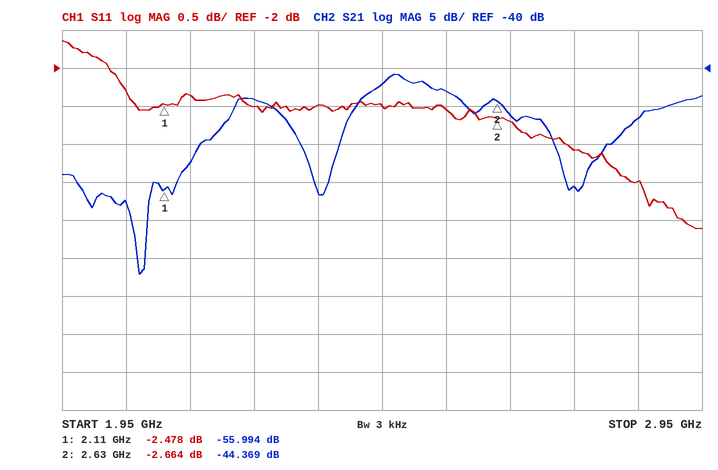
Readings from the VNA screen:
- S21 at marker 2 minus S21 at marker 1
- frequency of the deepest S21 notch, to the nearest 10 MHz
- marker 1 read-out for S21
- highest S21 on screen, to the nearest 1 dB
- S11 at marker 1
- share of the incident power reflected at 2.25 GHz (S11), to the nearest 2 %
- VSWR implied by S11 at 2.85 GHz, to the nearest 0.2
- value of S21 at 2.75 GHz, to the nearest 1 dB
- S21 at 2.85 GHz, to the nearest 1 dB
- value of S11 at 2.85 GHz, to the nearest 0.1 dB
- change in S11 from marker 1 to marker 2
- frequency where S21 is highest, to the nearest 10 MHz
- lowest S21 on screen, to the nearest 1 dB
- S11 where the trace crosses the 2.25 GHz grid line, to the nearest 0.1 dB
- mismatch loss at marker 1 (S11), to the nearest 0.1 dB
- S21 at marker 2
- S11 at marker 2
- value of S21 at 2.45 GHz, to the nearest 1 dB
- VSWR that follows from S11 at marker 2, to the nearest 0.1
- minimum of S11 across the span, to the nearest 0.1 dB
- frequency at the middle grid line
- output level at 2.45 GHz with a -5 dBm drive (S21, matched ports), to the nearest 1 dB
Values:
11.625 dB
2.07 GHz
-55.994 dB
-41 dB
-2.478 dB
56 %
5.0
-56 dB
-47 dB
-3.5 dB
-0.186 dB
2.47 GHz
-67 dB
-2.5 dB
3.6 dB
-44.369 dB
-2.664 dB
-42 dB
6.6
-4.1 dB
2.45 GHz
-47 dBm
